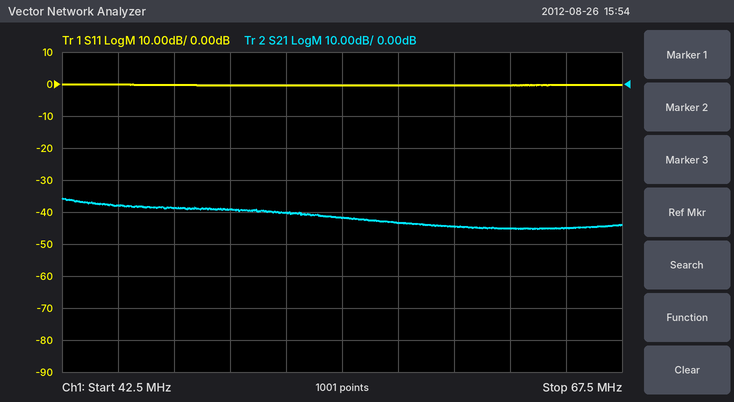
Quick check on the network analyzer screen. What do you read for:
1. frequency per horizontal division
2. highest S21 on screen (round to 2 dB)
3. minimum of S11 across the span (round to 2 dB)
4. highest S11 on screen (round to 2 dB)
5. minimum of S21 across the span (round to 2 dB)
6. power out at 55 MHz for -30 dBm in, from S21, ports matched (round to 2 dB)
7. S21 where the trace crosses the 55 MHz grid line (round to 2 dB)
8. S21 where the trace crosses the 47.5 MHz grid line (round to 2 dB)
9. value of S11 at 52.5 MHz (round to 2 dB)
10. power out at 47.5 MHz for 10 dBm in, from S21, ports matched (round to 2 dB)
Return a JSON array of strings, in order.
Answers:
["2.5 MHz", "-36 dB", "0 dB", "0 dB", "-46 dB", "-72 dBm", "-42 dB", "-38 dB", "0 dB", "-28 dBm"]
